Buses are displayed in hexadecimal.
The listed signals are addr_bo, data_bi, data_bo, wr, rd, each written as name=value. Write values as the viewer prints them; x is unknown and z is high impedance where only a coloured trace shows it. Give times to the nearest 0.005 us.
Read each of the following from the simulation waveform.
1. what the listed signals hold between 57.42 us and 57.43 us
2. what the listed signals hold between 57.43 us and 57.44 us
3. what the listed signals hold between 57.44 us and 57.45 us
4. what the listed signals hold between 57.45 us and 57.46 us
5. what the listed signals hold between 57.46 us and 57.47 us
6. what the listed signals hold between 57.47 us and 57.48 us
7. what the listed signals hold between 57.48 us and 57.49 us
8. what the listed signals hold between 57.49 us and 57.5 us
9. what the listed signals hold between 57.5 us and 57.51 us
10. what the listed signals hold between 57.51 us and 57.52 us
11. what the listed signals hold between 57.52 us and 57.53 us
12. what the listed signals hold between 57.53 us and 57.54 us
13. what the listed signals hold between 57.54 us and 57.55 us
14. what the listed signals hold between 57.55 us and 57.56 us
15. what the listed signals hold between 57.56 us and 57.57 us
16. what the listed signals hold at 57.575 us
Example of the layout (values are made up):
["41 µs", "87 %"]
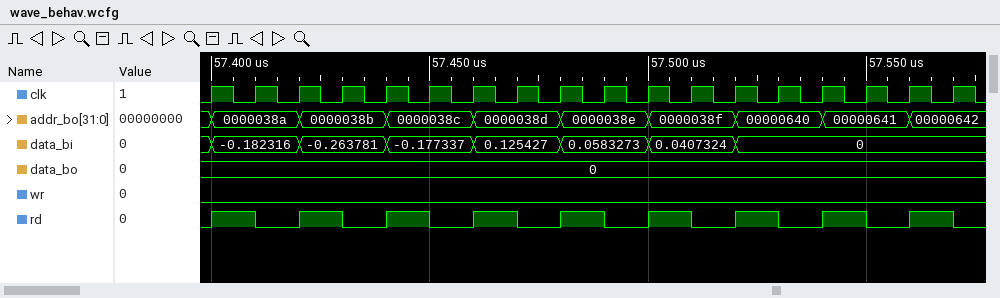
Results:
["addr_bo=0000038b, data_bi=-0.263781, data_bo=0, wr=0, rd=1", "addr_bo=0000038b, data_bi=-0.263781, data_bo=0, wr=0, rd=0", "addr_bo=0000038c, data_bi=-0.177337, data_bo=0, wr=0, rd=1", "addr_bo=0000038c, data_bi=-0.177337, data_bo=0, wr=0, rd=0", "addr_bo=0000038d, data_bi=0.125427, data_bo=0, wr=0, rd=1", "addr_bo=0000038d, data_bi=0.125427, data_bo=0, wr=0, rd=0", "addr_bo=0000038e, data_bi=0.0583273, data_bo=0, wr=0, rd=1", "addr_bo=0000038e, data_bi=0.0583273, data_bo=0, wr=0, rd=0", "addr_bo=0000038f, data_bi=0.0407324, data_bo=0, wr=0, rd=1", "addr_bo=0000038f, data_bi=0.0407324, data_bo=0, wr=0, rd=0", "addr_bo=00000640, data_bi=0, data_bo=0, wr=0, rd=1", "addr_bo=00000640, data_bi=0, data_bo=0, wr=0, rd=0", "addr_bo=00000641, data_bi=0, data_bo=0, wr=0, rd=1", "addr_bo=00000641, data_bi=0, data_bo=0, wr=0, rd=0", "addr_bo=00000642, data_bi=0, data_bo=0, wr=0, rd=1", "addr_bo=00000642, data_bi=0, data_bo=0, wr=0, rd=0"]
